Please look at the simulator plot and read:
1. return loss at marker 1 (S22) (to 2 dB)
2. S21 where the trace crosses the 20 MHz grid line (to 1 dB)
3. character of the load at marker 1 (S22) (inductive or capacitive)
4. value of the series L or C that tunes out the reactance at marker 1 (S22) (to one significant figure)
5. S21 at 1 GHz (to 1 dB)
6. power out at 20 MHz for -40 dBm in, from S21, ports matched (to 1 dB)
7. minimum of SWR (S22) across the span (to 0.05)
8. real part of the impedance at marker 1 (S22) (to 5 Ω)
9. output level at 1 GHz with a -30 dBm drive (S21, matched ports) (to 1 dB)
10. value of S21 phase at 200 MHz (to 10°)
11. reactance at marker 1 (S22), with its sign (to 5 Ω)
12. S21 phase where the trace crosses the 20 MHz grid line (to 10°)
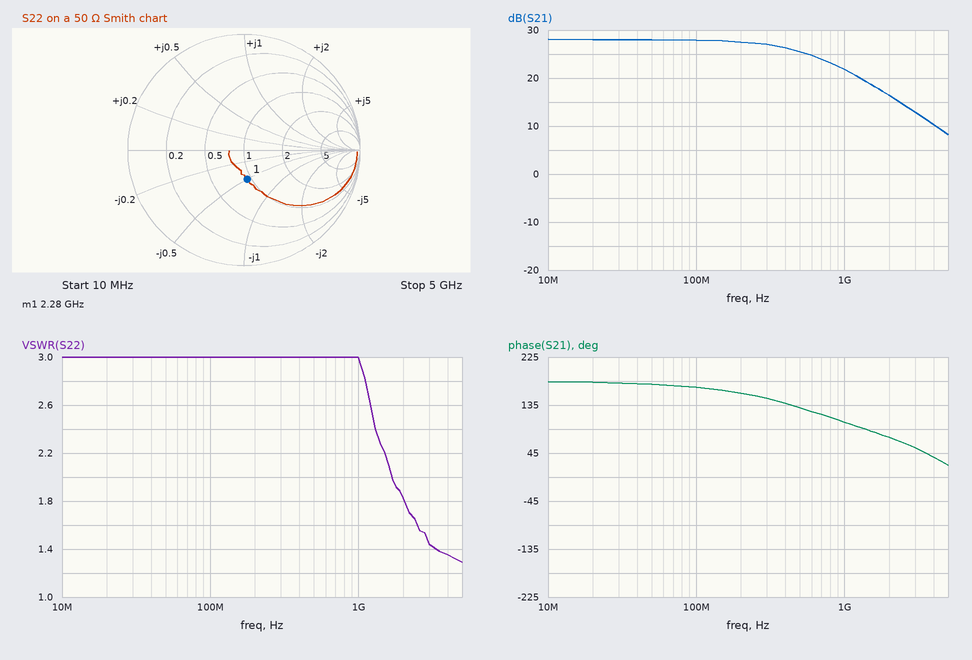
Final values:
12 dB
28 dB
capacitive
2 nH
22 dB
-12 dBm
1.30
45 Ω
-8 dBm
160°
-25 Ω
180°
